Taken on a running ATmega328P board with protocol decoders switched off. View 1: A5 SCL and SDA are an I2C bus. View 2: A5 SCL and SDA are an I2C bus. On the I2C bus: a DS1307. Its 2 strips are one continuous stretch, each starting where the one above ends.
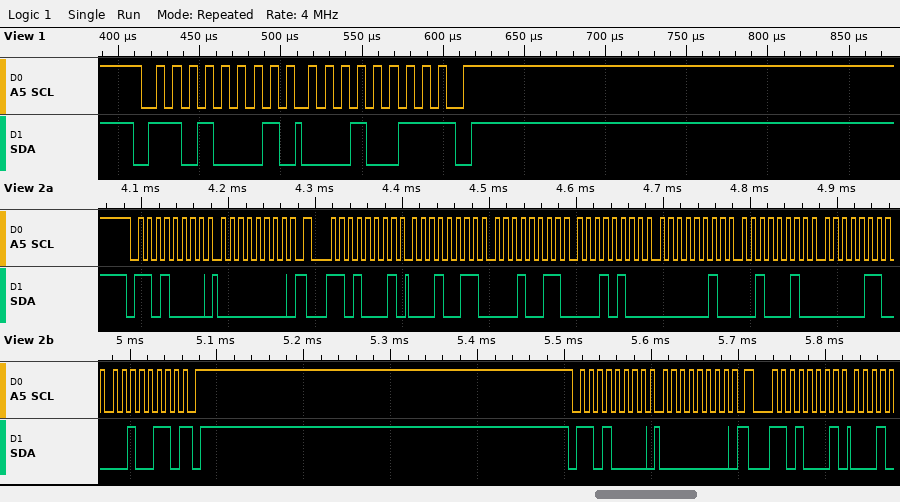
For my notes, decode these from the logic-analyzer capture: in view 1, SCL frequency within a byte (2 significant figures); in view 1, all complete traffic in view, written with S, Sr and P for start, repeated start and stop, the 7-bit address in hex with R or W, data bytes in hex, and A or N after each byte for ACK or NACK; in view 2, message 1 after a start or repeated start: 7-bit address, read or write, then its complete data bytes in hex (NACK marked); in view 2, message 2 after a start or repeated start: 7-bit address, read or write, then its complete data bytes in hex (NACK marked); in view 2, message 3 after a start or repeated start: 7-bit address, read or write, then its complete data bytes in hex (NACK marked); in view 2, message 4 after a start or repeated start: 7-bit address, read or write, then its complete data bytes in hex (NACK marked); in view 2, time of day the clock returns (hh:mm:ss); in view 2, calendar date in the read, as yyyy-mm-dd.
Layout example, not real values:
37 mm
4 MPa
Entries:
100 kHz
S 68R A 13 N P
0x68 write: 00
0x68 read: 13 13 14 02 22 06 26 NACK
0x68 write: 00
0x68 read
14:13:13
2026-06-22
